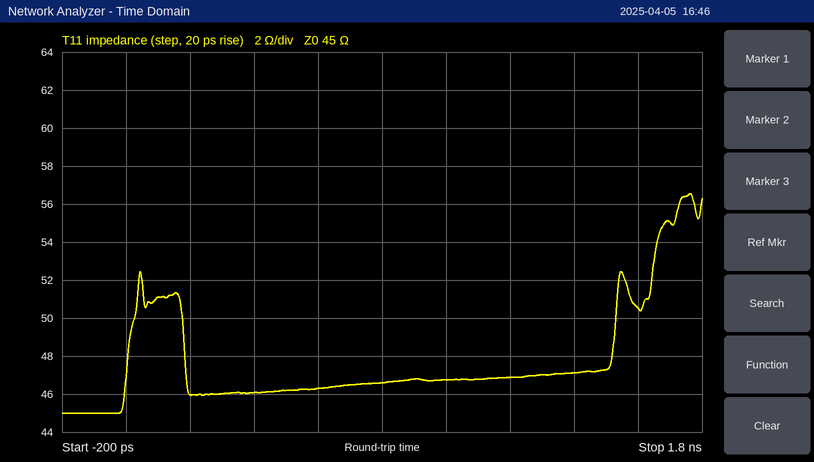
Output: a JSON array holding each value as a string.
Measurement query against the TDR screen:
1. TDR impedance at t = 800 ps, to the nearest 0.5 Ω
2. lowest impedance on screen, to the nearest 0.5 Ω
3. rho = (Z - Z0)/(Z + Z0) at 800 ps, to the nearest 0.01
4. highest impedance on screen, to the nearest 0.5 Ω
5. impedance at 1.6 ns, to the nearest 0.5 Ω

["46.5 Ω", "45.0 Ω", "+0.02", "56.5 Ω", "50.5 Ω"]
